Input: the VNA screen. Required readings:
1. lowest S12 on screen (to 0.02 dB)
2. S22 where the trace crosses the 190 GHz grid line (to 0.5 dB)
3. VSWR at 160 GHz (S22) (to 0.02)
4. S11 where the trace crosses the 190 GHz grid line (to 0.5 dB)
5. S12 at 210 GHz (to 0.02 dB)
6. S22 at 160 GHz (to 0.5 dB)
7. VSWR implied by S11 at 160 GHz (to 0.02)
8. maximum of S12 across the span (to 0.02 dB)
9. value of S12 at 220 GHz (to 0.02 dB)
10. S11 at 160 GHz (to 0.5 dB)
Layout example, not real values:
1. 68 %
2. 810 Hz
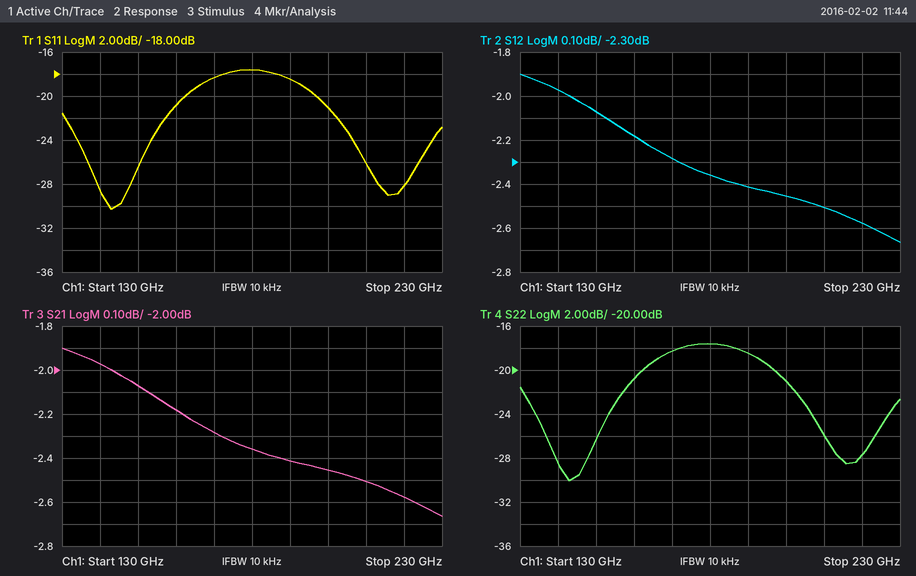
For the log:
1. -2.66 dB
2. -18.5 dB
3. 1.20
4. -18.5 dB
5. -2.50 dB
6. -21.0 dB
7. 1.20
8. -1.90 dB
9. -2.58 dB
10. -21.0 dB
